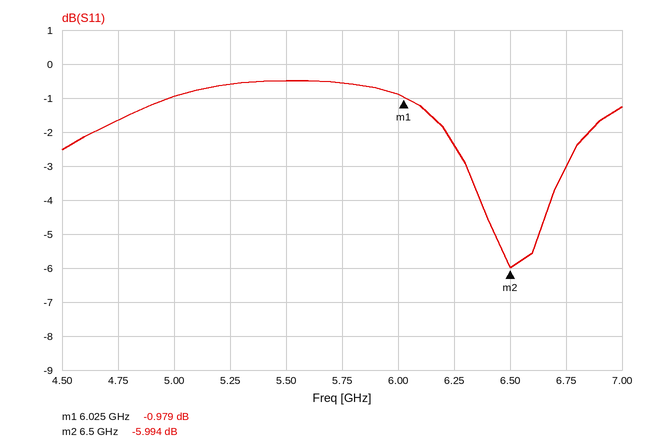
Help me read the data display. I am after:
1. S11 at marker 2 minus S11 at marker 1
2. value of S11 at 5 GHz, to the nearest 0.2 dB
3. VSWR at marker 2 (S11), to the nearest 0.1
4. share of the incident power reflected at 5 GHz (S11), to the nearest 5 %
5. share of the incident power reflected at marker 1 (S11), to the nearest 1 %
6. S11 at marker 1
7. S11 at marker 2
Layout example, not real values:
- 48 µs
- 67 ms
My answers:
- -5.015 dB
- -1.0 dB
- 3.0
- 80 %
- 80 %
- -0.979 dB
- -5.994 dB
